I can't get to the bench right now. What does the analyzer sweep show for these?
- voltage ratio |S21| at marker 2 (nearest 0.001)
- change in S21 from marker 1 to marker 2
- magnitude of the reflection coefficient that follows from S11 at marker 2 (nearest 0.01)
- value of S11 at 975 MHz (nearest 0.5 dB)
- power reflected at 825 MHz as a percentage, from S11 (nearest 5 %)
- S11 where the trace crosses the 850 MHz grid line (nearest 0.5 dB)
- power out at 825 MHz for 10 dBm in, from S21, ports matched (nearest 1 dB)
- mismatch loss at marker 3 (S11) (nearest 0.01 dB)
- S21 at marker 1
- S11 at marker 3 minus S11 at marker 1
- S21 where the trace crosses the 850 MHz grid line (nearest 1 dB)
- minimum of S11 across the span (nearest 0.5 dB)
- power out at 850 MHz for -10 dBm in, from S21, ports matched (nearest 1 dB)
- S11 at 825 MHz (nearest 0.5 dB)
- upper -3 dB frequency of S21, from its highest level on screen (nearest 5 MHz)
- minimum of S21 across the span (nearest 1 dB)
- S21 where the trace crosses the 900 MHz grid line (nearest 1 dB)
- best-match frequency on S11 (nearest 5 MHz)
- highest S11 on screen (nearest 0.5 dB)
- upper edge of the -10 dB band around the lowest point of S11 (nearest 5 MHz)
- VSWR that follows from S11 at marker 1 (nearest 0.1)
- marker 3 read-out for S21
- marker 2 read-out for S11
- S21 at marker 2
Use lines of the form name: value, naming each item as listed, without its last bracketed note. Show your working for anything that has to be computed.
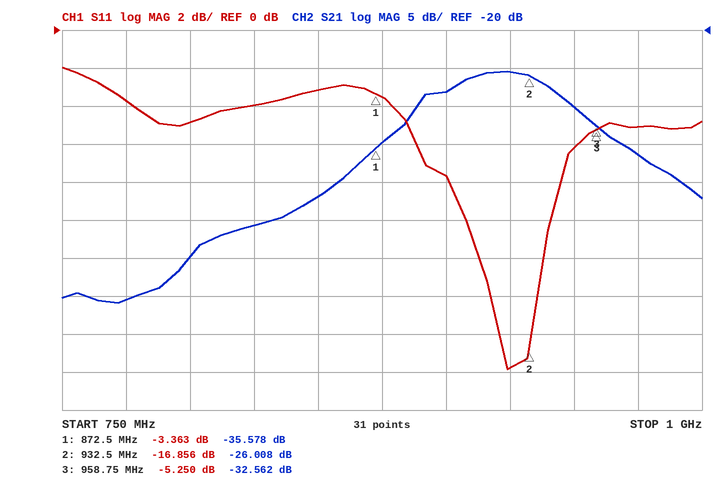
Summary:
voltage ratio |S21| at marker 2: 10^(-26.008/20) ≈ 0.050
change in S21 from marker 1 to marker 2: -26.008 − (-35.578) = 9.570 dB
magnitude of the reflection coefficient that follows from S11 at marker 2: 10^(-16.856/20) ≈ 0.14
value of S11 at 975 MHz: -5.0 dB
power reflected at 825 MHz as a percentage, from S11: 10^(-4/10) ≈ 40 %
S11 where the trace crosses the 850 MHz grid line: -3.0 dB
power out at 825 MHz for 10 dBm in, from S21, ports matched: 10 dBm + (-46 dB) = -36 dBm
mismatch loss at marker 3 (S11): −10 log10(1 − 10^(-5.25/10)) ≈ 1.54 dB
S21 at marker 1: -35.578 dB
S11 at marker 3 minus S11 at marker 1: -5.25 − (-3.363) = -1.887 dB
S21 where the trace crosses the 850 MHz grid line: -42 dB
minimum of S11 across the span: -18.0 dB
power out at 850 MHz for -10 dBm in, from S21, ports matched: -10 dBm + (-42 dB) = -52 dBm
S11 at 825 MHz: -4.0 dB
upper -3 dB frequency of S21, from its highest level on screen: 945 MHz
minimum of S21 across the span: -56 dB
S21 where the trace crosses the 900 MHz grid line: -28 dB
best-match frequency on S11: 925 MHz
highest S11 on screen: -2.0 dB
upper edge of the -10 dB band around the lowest point of S11: 940 MHz
VSWR that follows from S11 at marker 1: (1 + 0.6790)/(1 − 0.6790) ≈ 5.2
marker 3 read-out for S21: -32.562 dB
marker 2 read-out for S11: -16.856 dB
S21 at marker 2: -26.008 dB
